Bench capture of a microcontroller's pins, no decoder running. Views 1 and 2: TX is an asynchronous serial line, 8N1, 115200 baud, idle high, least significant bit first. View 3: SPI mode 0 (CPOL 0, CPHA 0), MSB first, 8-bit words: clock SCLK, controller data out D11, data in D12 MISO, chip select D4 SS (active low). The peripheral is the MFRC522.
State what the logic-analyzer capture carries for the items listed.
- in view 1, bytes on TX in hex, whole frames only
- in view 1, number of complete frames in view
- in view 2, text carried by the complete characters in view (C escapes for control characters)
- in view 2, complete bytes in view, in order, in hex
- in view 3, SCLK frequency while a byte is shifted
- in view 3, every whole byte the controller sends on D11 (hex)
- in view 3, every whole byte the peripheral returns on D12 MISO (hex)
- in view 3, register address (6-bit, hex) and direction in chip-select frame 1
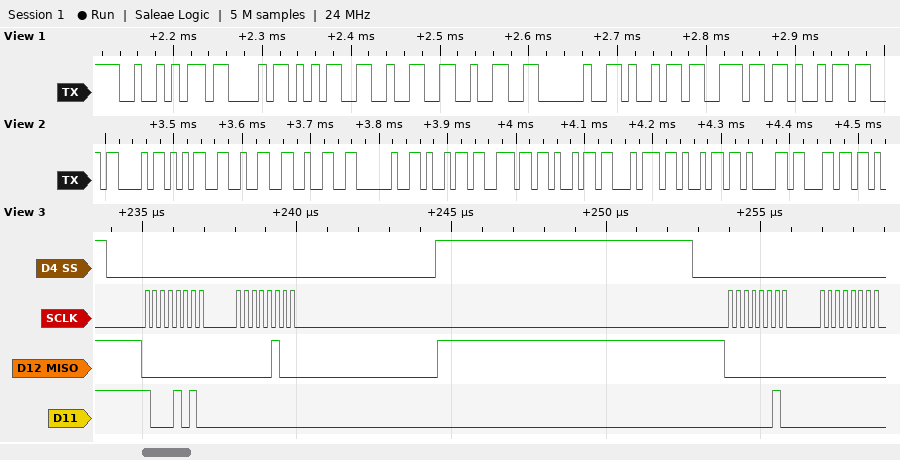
52 43 35 32 32 20 69 6E 69
9
"C522 initial"
43 35 32 32 20 69 6E 69 74 69 61 6C
4 MHz
0x8A 0x00 0x02 0x00
0x00 0x04 0x00 0x00
0x05 read
